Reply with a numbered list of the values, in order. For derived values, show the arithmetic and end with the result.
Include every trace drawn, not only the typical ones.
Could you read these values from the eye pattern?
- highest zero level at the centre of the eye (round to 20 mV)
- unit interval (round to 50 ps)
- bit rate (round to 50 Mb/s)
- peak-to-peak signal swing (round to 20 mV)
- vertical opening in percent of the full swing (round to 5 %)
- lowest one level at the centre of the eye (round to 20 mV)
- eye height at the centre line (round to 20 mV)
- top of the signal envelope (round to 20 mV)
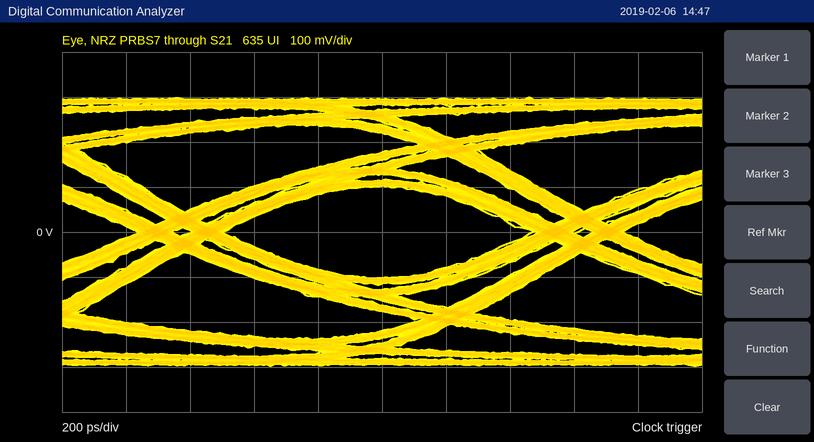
1. -100 mV
2. 1.25 ns
3. 800 Mb/s
4. 600 mV
5. 200 mV / 600 mV ≈ 33.3 %, so 35 % to the nearest 5 %
6. 100 mV
7. 200 mV
8. 300 mV
